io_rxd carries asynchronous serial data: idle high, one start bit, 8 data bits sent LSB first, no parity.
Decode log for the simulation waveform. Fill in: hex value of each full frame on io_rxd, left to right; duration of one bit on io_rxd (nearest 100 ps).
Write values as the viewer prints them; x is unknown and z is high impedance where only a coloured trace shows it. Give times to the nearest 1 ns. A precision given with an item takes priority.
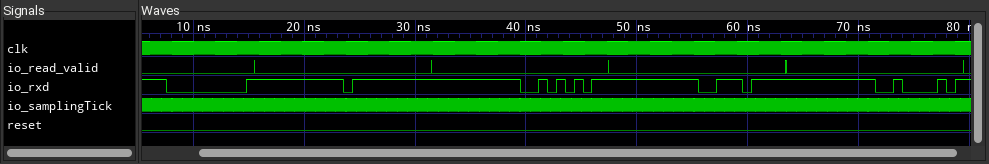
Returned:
00, FF, AA, EE, 42
800 ps
